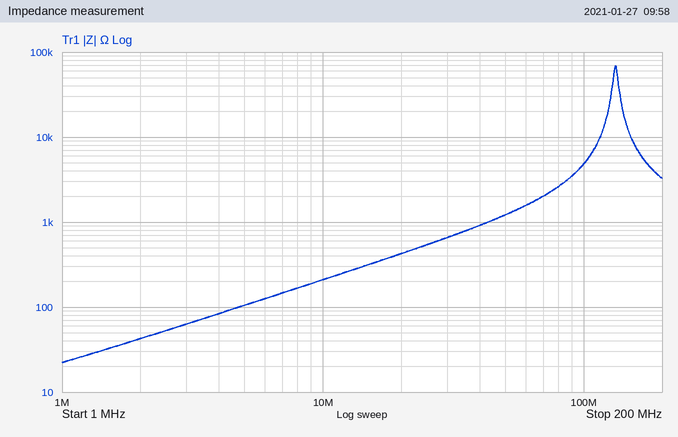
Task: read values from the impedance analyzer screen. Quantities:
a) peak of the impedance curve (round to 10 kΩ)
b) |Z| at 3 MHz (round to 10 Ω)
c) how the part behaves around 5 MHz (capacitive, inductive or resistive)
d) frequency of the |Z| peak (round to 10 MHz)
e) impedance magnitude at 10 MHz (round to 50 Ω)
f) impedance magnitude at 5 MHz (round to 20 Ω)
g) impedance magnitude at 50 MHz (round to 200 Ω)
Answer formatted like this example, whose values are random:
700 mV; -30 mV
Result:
70 kΩ; 60 Ω; inductive; 130 MHz; 200 Ω; 100 Ω; 1.2 kΩ
